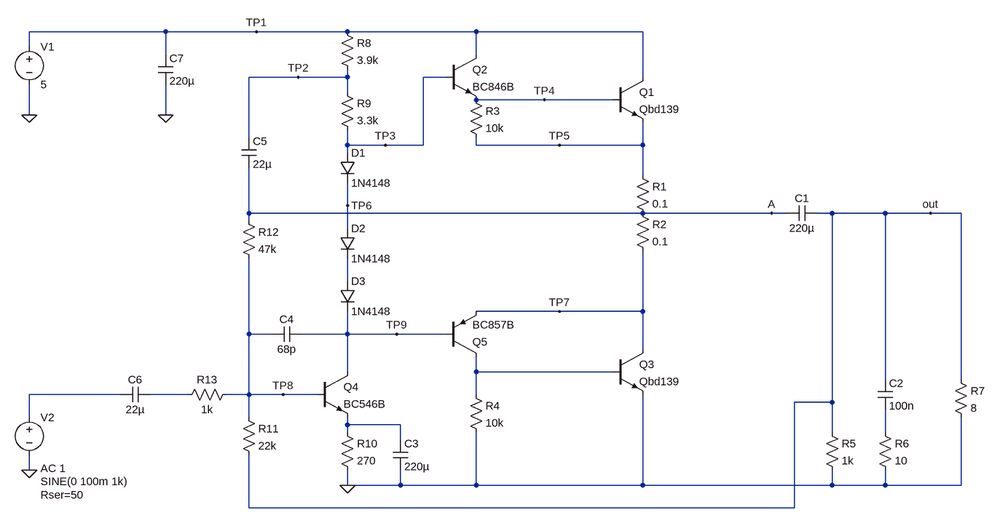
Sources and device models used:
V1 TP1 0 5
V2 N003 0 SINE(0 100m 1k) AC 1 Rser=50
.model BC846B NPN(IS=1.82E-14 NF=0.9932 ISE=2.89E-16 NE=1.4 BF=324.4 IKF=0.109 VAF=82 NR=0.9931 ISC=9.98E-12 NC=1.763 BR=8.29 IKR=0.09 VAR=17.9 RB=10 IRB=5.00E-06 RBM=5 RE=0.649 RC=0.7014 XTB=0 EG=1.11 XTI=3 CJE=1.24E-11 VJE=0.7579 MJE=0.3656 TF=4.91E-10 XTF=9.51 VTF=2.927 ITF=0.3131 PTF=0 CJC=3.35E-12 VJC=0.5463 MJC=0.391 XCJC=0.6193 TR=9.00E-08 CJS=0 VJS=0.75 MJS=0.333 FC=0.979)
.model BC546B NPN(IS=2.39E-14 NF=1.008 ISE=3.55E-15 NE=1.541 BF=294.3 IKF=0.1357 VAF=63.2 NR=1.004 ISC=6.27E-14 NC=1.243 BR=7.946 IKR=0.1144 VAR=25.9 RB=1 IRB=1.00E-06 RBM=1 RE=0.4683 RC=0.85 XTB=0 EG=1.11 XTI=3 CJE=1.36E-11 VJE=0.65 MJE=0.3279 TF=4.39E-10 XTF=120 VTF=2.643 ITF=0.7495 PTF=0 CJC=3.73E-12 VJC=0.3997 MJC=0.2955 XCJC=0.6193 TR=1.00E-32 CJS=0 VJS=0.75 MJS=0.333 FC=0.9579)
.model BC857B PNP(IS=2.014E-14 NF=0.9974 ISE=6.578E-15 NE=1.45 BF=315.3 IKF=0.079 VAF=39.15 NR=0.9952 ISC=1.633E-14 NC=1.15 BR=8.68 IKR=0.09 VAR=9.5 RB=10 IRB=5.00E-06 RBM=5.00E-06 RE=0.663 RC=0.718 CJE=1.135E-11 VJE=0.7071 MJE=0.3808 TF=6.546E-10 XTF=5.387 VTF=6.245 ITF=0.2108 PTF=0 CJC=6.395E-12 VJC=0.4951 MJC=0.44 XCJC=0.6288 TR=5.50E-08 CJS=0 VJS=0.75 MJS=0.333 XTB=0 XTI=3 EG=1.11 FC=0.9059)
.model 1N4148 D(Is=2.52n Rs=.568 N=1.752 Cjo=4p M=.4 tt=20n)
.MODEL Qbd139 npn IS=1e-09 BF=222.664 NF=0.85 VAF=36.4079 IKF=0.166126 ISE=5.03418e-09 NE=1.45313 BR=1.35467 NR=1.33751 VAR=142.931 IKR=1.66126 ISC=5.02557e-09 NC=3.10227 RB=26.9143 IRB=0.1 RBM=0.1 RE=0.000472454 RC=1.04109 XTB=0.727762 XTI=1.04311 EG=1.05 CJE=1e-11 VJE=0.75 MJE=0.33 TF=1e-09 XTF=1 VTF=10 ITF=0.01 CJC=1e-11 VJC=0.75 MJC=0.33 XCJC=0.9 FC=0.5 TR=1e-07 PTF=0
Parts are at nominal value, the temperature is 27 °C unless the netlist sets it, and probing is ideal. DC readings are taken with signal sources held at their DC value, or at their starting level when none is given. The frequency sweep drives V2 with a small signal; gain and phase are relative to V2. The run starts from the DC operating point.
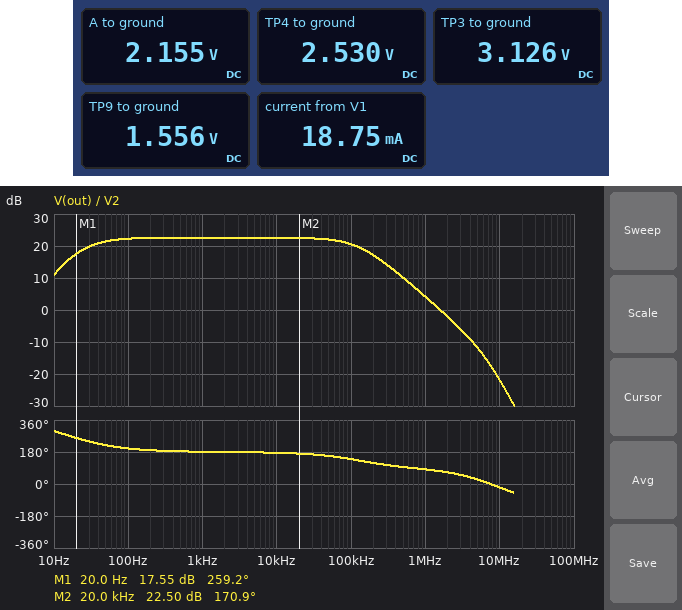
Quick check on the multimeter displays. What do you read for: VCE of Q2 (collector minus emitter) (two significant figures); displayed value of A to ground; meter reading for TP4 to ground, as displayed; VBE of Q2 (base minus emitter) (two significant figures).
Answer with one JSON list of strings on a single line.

["2.5 V", "2.155 V", "2.530 V", "600 mV"]
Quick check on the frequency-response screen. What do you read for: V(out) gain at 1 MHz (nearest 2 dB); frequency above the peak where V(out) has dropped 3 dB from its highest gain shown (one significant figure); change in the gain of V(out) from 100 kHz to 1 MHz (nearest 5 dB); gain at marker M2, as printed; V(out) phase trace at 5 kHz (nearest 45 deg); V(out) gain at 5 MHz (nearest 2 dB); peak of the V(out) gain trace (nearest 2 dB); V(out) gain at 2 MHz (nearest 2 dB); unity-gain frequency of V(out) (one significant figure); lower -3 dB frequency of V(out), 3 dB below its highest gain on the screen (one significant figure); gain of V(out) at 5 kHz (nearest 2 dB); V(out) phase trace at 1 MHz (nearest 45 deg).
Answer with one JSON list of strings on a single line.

["4 dB", "100 kHz", "-15 dB", "22.50 dB", "180 deg", "-12 dB", "22 dB", "-2 dB", "2 MHz", "30 Hz", "22 dB", "90 deg"]
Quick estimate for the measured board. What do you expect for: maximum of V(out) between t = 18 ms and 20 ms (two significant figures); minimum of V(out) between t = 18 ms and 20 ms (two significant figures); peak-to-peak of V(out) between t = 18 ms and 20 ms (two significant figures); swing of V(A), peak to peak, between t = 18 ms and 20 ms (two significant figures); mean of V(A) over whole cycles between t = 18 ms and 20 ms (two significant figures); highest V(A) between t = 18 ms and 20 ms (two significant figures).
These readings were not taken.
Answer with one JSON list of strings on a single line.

["1.3 V", "-1.3 V", "2.6 V", "2.6 V", "2.1 V", "3.5 V"]
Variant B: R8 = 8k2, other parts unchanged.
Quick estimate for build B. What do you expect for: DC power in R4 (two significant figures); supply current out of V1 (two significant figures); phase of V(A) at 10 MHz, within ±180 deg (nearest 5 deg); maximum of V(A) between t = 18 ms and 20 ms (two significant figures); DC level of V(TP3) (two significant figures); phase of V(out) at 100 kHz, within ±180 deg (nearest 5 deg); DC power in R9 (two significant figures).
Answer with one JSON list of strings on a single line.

["12 µW", "8.1 mA", "-40 deg", "3.3 V", "3.0 V", "135 deg", "100 µW"]
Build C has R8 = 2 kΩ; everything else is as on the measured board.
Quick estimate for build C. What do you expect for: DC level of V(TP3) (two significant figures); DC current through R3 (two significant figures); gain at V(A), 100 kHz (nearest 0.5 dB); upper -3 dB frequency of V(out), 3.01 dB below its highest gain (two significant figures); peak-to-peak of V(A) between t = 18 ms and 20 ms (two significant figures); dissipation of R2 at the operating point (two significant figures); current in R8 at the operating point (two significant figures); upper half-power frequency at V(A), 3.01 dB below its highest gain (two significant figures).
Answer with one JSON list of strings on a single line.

["3.2 V", "39 µA", "21.0 dB", "130 kHz", "2.7 V", "83 µW", "330 µA", "49 Hz"]
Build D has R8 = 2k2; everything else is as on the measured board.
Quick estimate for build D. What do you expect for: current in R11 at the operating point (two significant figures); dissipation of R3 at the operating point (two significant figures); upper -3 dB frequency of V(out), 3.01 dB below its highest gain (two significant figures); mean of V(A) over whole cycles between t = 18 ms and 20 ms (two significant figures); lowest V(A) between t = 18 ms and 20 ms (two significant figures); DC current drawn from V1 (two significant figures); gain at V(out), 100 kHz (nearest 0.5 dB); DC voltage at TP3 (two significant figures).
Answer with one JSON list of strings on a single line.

["32 µA", "15 µW", "130 kHz", "2.2 V", "870 mV", "28 mA", "21.0 dB", "3.2 V"]
